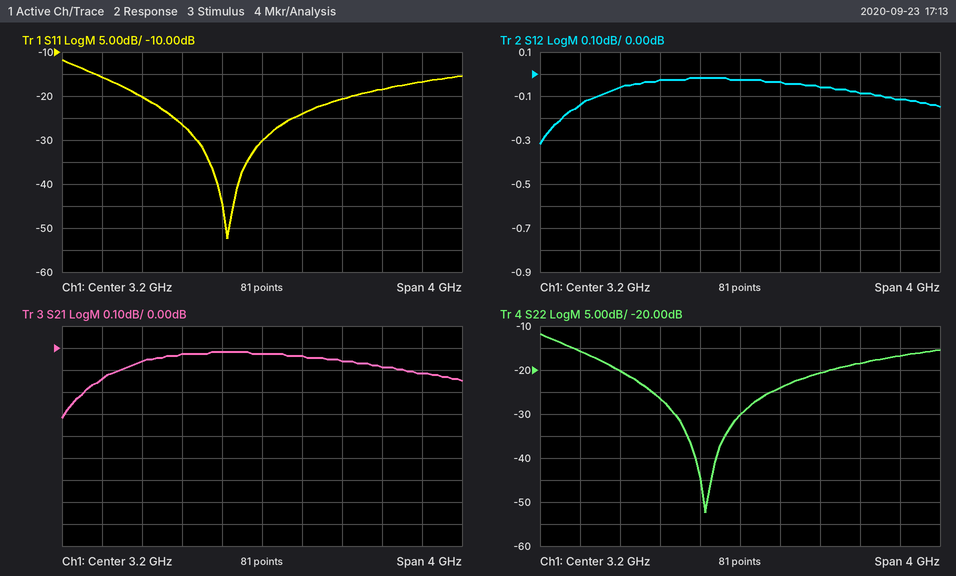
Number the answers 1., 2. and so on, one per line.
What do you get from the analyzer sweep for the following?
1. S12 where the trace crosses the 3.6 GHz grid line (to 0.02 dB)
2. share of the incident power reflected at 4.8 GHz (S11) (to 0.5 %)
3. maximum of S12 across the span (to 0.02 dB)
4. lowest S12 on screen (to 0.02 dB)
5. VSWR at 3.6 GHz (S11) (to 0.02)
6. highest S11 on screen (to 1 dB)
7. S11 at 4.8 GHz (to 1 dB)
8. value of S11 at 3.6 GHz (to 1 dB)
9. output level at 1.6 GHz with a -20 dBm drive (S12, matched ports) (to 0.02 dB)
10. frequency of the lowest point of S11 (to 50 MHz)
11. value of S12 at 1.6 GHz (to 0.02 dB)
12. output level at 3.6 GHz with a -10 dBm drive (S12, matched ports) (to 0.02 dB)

1. -0.04 dB
2. 2.0 %
3. -0.02 dB
4. -0.32 dB
5. 1.14
6. -12 dB
7. -17 dB
8. -24 dB
9. -20.14 dBm
10. 2.85 GHz
11. -0.14 dB
12. -10.04 dBm
